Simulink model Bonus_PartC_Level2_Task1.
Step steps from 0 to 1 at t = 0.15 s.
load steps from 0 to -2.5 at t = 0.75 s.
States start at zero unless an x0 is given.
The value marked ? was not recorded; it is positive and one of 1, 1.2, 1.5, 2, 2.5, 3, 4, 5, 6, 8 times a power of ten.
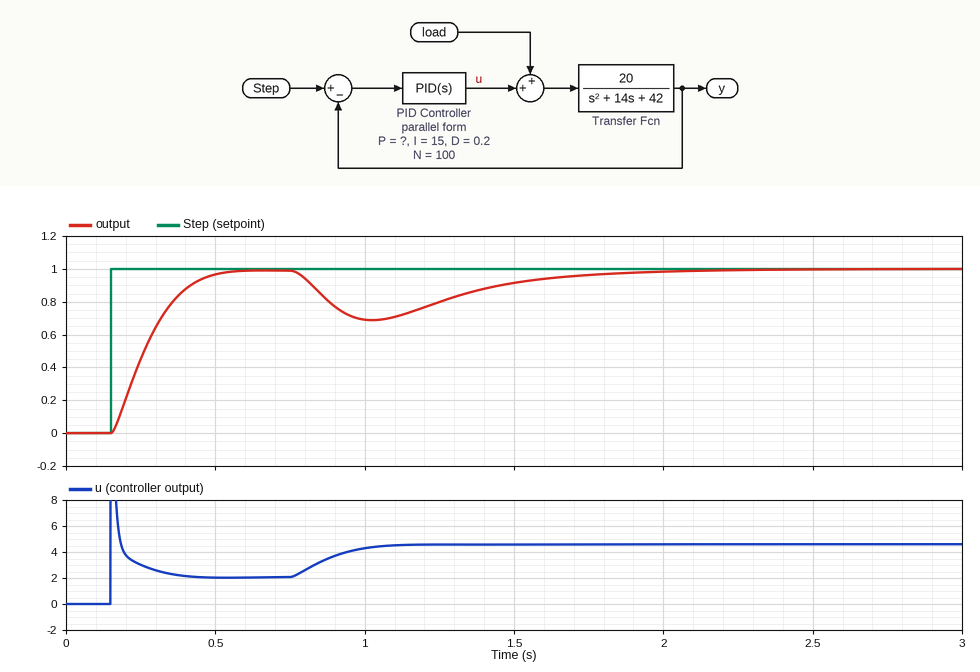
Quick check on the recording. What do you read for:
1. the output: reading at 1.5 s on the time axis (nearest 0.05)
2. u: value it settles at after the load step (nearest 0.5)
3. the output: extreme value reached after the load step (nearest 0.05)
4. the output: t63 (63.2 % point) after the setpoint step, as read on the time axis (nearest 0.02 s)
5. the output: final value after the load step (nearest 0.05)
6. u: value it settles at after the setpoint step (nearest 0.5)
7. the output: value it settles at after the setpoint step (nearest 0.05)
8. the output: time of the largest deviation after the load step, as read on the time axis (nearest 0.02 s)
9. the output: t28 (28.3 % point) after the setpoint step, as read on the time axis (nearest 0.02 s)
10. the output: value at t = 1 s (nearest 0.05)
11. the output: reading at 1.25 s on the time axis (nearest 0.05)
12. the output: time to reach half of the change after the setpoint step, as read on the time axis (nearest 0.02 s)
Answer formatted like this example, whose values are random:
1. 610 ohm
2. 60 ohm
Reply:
1. 0.90
2. 4.5
3. 0.70
4. 0.30 s
5. 1.00
6. 2.0
7. 1.00
8. 1.02 s
9. 0.22 s
10. 0.70
11. 0.80
12. 0.26 s
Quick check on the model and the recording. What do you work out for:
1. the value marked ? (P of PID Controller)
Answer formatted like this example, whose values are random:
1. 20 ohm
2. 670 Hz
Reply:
1. 5
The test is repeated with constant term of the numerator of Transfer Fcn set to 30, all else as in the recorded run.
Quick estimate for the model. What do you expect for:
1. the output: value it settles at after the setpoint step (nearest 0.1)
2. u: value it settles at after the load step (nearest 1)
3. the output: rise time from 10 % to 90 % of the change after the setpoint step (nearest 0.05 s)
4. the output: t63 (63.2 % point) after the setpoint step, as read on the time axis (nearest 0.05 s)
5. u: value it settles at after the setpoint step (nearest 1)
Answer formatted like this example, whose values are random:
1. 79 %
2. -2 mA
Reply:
1. 1.0
2. 4
3. 0.15 s
4. 0.25 s
5. 1
